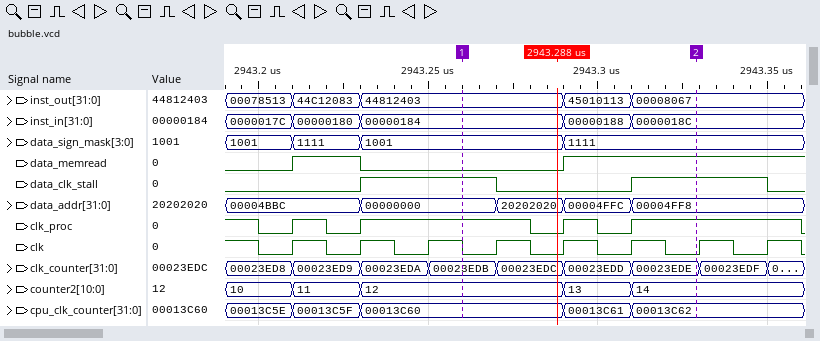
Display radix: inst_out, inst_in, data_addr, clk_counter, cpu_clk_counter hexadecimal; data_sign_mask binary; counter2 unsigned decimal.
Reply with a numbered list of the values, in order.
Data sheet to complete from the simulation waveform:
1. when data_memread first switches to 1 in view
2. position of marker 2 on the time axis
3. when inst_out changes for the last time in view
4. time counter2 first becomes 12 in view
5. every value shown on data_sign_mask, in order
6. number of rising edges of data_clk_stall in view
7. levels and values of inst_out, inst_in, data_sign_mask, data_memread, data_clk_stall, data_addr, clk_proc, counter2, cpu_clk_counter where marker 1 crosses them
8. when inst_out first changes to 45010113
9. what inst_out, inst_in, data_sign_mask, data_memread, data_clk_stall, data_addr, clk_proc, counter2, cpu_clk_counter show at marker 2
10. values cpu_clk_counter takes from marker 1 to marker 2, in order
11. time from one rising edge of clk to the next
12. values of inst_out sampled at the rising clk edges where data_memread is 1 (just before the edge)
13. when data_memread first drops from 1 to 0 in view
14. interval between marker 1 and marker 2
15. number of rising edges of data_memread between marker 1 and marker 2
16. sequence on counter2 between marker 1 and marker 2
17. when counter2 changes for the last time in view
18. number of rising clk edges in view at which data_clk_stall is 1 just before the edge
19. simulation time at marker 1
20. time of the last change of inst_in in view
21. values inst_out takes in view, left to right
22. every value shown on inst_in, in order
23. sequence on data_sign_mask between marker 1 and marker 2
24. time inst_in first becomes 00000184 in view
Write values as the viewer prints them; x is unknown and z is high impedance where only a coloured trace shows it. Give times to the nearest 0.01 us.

1. 2943.21 us
2. 2943.33 us
3. 2943.31 us
4. 2943.23 us
5. 1001, 1111, 1001, 1111
6. 2
7. inst_out=44812403, inst_in=00000184, data_sign_mask=1001, data_memread=0, data_clk_stall=1, data_addr=00000000, clk_proc=1, counter2=12, cpu_clk_counter=00013C60
8. 2943.29 us
9. inst_out=00008067, inst_in=0000018C, data_sign_mask=1111, data_memread=1, data_clk_stall=1, data_addr=00004FF8, clk_proc=1, counter2=14, cpu_clk_counter=00013C62
10. 00013C60, 00013C61, 00013C62
11. 0.02 us
12. 44C12083, 45010113, 00008067, 00008067
13. 2943.23 us
14. 0.07 us
15. 1
16. 12, 13, 14
17. 2943.31 us
18. 4
19. 2943.26 us
20. 2943.31 us
21. 00078513, 44C12083, 44812403, 45010113, 00008067
22. 0000017C, 00000180, 00000184, 00000188, 0000018C
23. 1001, 1111
24. 2943.23 us
